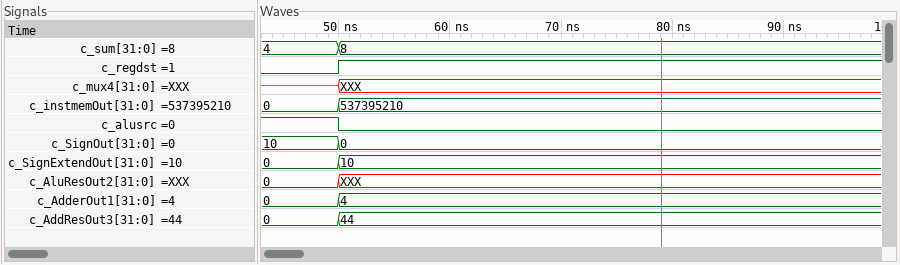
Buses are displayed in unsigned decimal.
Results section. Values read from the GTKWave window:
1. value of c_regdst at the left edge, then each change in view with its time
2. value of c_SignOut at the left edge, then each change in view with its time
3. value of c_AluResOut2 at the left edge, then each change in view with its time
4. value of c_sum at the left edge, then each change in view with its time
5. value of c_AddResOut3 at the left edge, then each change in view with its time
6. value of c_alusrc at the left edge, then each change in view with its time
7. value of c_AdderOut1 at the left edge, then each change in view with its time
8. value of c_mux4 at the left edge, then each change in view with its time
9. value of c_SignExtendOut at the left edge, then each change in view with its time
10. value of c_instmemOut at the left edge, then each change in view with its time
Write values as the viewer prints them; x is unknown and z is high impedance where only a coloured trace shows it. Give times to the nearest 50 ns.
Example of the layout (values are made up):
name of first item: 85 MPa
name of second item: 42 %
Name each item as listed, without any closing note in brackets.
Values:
value of c_regdst at the left edge, then each change in view with its time: 0, 1 at 50 ns
value of c_SignOut at the left edge, then each change in view with its time: 10, 0 at 50 ns
value of c_AluResOut2 at the left edge, then each change in view with its time: 0, XXX at 50 ns
value of c_sum at the left edge, then each change in view with its time: 4, 8 at 50 ns
value of c_AddResOut3 at the left edge, then each change in view with its time: 0, 44 at 50 ns
value of c_alusrc at the left edge, then each change in view with its time: 1, 0 at 50 ns
value of c_AdderOut1 at the left edge, then each change in view with its time: 0, 4 at 50 ns
value of c_mux4 at the left edge, then each change in view with its time: z, XXX at 50 ns
value of c_SignExtendOut at the left edge, then each change in view with its time: 0, 10 at 50 ns
value of c_instmemOut at the left edge, then each change in view with its time: 0, 537395210 at 50 ns
